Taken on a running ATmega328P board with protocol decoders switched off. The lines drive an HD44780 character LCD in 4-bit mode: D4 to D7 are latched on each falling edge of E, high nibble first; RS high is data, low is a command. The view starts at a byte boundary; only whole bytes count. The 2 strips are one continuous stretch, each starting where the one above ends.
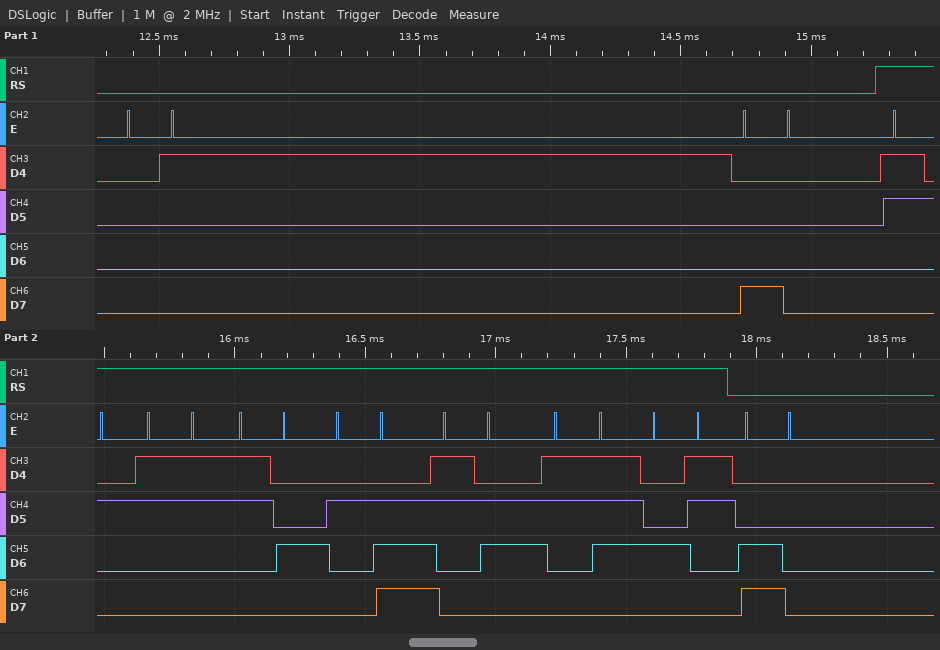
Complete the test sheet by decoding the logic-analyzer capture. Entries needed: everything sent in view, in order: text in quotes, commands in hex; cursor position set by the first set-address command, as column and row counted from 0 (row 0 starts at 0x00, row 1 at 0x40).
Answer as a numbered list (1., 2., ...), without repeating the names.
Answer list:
1. 0x01 0x80 "234.67C" 0xC0
2. column 0, row 0
